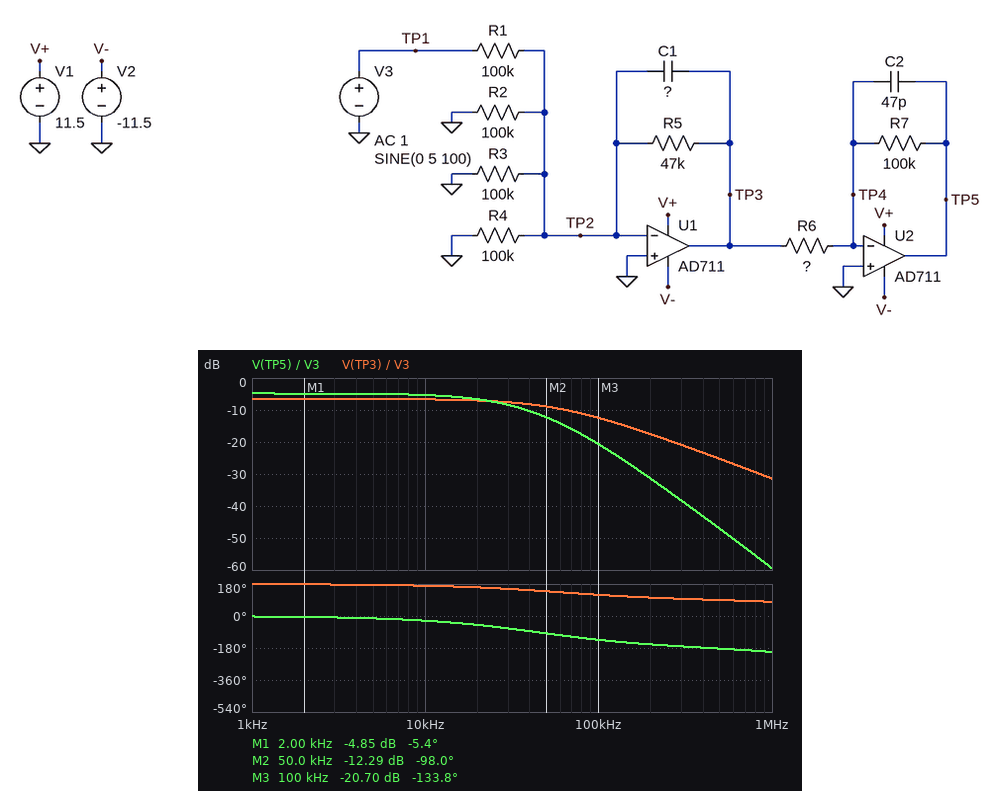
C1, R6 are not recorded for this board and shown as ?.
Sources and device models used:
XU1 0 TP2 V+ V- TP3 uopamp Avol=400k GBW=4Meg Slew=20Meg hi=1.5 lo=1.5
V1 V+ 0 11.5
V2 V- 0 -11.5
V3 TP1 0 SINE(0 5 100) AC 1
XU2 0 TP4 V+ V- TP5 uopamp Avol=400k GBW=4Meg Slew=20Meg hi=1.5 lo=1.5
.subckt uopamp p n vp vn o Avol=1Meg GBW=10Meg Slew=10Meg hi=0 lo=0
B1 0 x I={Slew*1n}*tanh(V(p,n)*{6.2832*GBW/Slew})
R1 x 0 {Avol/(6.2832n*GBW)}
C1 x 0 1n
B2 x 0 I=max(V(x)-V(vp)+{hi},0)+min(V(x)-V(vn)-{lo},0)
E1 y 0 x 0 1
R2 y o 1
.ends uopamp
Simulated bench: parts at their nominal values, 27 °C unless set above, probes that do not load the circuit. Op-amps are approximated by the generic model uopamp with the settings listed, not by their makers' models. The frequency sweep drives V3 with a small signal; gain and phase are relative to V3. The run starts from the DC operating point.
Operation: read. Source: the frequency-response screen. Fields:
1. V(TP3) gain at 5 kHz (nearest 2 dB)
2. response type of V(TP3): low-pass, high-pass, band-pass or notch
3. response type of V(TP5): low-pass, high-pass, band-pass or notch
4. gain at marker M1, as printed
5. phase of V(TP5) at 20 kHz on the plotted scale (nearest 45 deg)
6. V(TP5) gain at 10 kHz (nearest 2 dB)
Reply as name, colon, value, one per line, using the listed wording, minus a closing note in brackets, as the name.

V(TP3) gain at 5 kHz: -6 dB
response type of V(TP3): low-pass, high-pass, band-pass or notch: low-pass
response type of V(TP5): low-pass, high-pass, band-pass or notch: low-pass
gain at marker M1, as printed: -4.85 dB
phase of V(TP5) at 20 kHz on the plotted scale: -45 deg
V(TP5) gain at 10 kHz: -6 dB
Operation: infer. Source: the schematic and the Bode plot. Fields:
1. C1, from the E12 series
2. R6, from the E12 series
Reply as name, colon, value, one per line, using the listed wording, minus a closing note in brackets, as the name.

C1, from the E12 series: 56 pF
R6, from the E12 series: 82 kΩ
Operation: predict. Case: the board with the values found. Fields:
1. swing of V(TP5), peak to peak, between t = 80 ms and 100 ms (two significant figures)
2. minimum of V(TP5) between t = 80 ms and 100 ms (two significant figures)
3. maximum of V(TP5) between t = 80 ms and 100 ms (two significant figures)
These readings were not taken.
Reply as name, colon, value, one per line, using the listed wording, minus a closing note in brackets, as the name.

swing of V(TP5), peak to peak, between t = 80 ms and 100 ms: 5.7 V
minimum of V(TP5) between t = 80 ms and 100 ms: -2.9 V
maximum of V(TP5) between t = 80 ms and 100 ms: 2.9 V
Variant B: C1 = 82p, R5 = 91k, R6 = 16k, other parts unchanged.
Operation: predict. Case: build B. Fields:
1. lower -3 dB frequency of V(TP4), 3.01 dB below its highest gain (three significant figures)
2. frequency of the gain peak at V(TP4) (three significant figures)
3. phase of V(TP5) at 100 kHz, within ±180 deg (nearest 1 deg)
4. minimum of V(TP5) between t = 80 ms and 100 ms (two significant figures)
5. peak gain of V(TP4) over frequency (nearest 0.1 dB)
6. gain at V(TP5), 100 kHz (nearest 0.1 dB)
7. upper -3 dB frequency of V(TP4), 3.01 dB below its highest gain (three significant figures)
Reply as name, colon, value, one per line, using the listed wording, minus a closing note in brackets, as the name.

lower -3 dB frequency of V(TP4), 3.01 dB below its highest gain: 10.6 kHz
frequency of the gain peak at V(TP4): 25.9 kHz
phase of V(TP5) at 100 kHz, within ±180 deg: -153 deg
minimum of V(TP5) between t = 80 ms and 100 ms: -10 V
peak gain of V(TP4) over frequency: -34.9 dB
gain at V(TP5), 100 kHz: -9.0 dB
upper -3 dB frequency of V(TP4), 3.01 dB below its highest gain: 63.6 kHz
